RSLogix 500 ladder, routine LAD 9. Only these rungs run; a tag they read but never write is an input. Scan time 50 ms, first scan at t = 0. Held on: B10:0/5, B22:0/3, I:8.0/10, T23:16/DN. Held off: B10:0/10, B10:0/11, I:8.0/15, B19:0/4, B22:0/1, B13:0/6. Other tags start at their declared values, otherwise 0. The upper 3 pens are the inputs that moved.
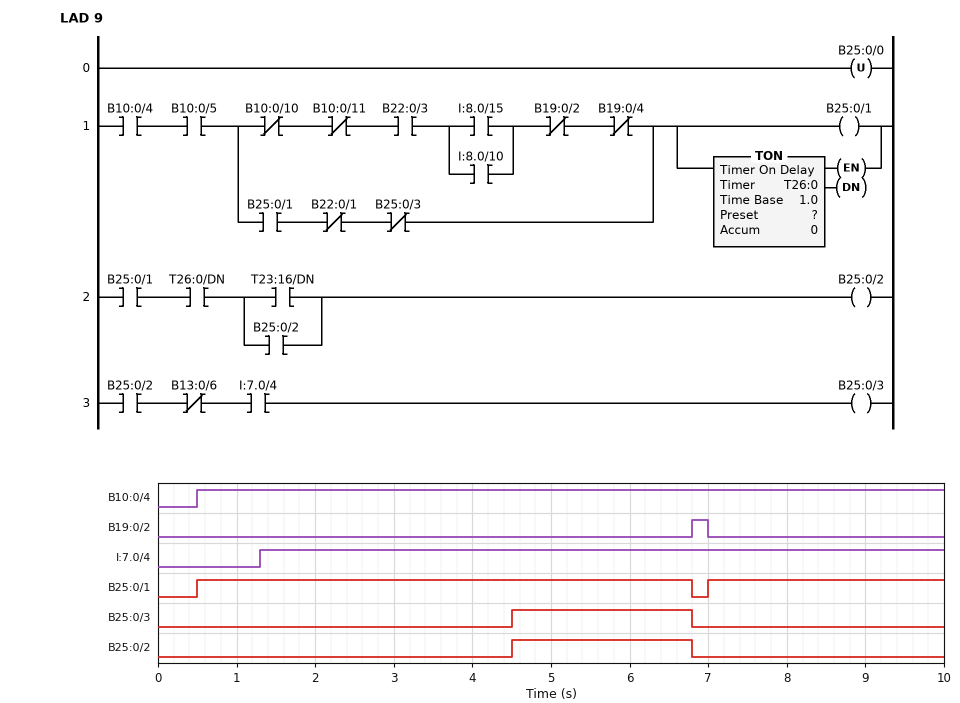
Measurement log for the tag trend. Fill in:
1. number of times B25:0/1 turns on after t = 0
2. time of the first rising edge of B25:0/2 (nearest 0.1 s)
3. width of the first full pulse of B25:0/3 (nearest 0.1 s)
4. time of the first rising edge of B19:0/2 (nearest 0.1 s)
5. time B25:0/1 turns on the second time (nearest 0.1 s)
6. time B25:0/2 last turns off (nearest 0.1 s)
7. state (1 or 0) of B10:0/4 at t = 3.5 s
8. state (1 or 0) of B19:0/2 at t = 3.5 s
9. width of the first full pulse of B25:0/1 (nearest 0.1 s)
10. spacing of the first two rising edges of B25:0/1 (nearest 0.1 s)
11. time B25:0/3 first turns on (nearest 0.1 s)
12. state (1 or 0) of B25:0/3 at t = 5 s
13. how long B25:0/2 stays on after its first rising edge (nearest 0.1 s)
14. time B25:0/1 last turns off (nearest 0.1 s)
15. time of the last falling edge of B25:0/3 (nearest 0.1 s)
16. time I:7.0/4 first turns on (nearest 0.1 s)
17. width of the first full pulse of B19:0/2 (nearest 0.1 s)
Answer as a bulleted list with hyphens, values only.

- 2
- 4.5 s
- 2.3 s
- 6.8 s
- 7.0 s
- 6.8 s
- 1
- 0
- 6.3 s
- 6.5 s
- 4.5 s
- 1
- 2.3 s
- 6.8 s
- 6.8 s
- 1.3 s
- 0.2 s
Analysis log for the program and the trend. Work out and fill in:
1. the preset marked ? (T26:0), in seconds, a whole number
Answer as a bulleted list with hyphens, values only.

- 4 s
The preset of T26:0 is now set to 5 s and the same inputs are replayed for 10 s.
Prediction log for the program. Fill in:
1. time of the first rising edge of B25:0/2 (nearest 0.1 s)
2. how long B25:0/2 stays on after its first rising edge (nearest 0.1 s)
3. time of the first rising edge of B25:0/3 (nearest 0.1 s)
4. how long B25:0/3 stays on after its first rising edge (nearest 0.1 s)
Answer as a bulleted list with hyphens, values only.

- 5.5 s
- 1.3 s
- 5.5 s
- 1.3 s
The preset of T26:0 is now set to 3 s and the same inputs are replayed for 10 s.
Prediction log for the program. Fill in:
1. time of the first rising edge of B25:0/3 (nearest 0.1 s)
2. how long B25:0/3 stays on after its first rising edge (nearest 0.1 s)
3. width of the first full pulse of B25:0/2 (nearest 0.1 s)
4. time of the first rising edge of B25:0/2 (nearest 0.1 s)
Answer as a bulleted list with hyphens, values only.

- 3.5 s
- 3.3 s
- 3.3 s
- 3.5 s
